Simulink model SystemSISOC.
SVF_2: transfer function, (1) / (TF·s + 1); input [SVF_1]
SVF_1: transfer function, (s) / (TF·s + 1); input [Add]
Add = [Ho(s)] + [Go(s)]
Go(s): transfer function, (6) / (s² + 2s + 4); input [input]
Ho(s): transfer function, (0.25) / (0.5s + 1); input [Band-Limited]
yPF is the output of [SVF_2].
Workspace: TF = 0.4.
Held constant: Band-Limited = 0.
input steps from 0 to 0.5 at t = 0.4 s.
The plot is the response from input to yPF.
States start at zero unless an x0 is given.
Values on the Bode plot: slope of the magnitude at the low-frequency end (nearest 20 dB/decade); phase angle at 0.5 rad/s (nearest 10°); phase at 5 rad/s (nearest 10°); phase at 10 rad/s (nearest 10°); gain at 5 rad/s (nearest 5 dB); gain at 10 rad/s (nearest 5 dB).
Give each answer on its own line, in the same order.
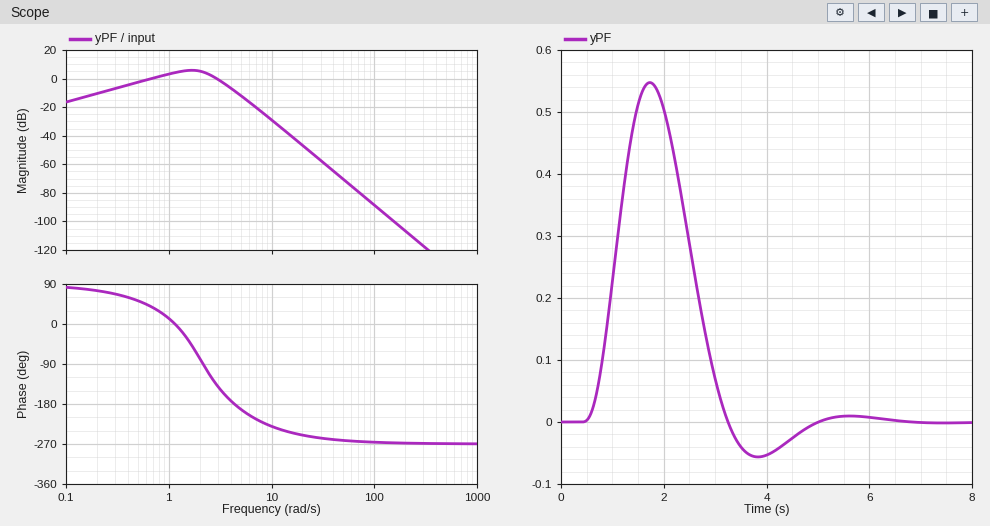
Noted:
20 dB/decade
50°
-190°
-230°
-10 dB
-30 dB
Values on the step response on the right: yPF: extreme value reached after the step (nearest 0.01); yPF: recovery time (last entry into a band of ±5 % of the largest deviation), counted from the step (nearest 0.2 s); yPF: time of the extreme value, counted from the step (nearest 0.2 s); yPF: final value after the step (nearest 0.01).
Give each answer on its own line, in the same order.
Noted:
0.55
4.0 s
1.4 s
0.00
